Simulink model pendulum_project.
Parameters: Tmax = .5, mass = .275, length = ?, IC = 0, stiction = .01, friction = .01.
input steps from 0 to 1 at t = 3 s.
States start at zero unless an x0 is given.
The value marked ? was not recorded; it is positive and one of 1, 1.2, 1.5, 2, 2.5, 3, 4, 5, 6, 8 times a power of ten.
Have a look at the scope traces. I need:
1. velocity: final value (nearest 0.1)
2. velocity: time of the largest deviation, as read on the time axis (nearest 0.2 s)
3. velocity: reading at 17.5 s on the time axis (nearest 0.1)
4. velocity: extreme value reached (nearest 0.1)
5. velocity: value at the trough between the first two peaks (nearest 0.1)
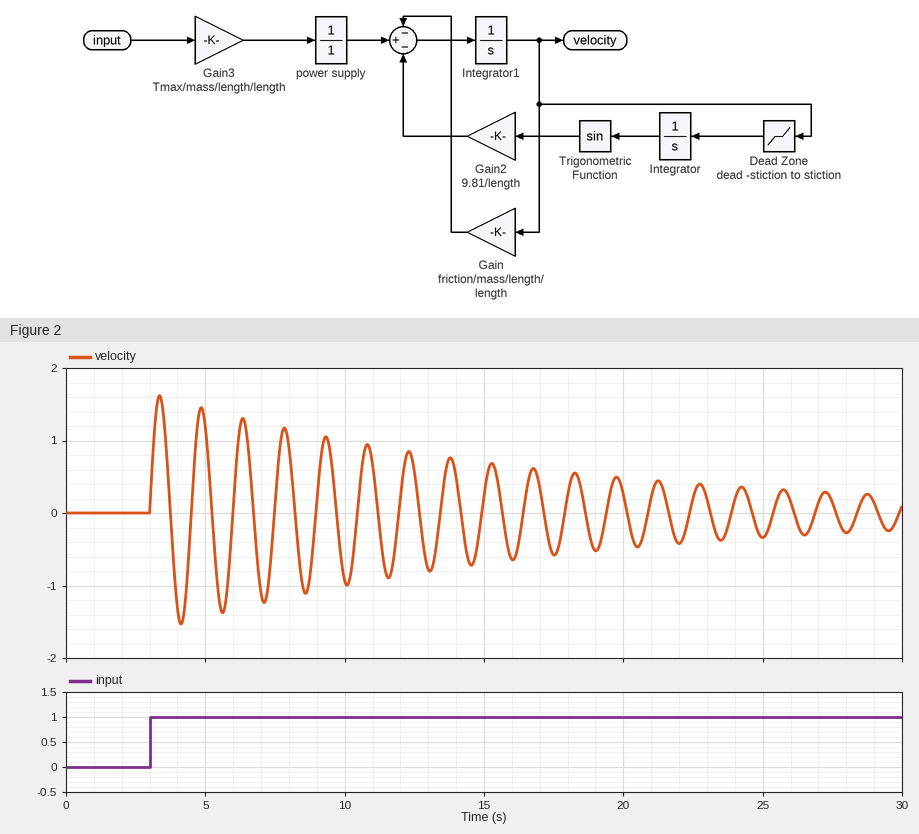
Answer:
0.0
3.4 s
-0.6
1.6
-1.5
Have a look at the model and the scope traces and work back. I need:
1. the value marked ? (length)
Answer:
0.5
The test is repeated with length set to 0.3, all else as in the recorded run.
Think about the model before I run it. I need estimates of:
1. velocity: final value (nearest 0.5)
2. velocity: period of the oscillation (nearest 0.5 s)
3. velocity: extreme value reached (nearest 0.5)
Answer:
0.0
1.5 s
3.5
